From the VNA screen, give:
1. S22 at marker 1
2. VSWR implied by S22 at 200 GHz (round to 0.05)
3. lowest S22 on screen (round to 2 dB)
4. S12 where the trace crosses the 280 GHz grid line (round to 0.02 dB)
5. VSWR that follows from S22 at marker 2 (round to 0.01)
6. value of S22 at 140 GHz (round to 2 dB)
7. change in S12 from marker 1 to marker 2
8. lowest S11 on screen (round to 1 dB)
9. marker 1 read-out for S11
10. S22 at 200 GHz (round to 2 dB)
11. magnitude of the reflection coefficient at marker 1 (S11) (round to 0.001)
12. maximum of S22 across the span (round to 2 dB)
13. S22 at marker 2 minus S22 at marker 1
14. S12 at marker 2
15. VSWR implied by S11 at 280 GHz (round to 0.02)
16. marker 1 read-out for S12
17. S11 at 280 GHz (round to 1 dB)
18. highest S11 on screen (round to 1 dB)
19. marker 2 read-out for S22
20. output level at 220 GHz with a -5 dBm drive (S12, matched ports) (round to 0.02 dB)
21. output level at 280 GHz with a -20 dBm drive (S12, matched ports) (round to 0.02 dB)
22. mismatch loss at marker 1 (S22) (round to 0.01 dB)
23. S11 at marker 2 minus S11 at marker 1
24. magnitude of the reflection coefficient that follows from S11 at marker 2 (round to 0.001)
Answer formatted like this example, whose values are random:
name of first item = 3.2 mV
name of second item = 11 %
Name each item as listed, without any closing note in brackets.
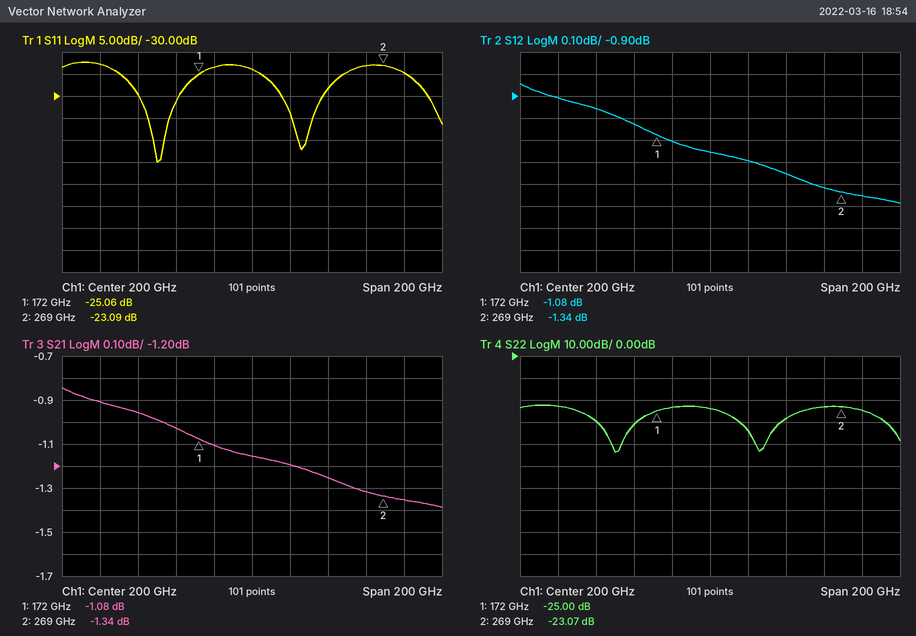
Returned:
S22 at marker 1 = -25.00 dB
VSWR implied by S22 at 200 GHz = 1.15
lowest S22 on screen = -44 dB
S12 where the trace crosses the 280 GHz grid line = -1.36 dB
VSWR that follows from S22 at marker 2 = 1.15
value of S22 at 140 GHz = -30 dB
change in S12 from marker 1 to marker 2 = -0.26 dB
lowest S11 on screen = -45 dB
marker 1 read-out for S11 = -25.06 dB
S22 at 200 GHz = -24 dB
magnitude of the reflection coefficient at marker 1 (S11) = 0.056
maximum of S22 across the span = -22 dB
S22 at marker 2 minus S22 at marker 1 = 1.93 dB
S12 at marker 2 = -1.34 dB
VSWR implied by S11 at 280 GHz = 1.12
marker 1 read-out for S12 = -1.08 dB
S11 at 280 GHz = -25 dB
highest S11 on screen = -22 dB
marker 2 read-out for S22 = -23.07 dB
output level at 220 GHz with a -5 dBm drive (S12, matched ports) = -6.20 dBm
output level at 280 GHz with a -20 dBm drive (S12, matched ports) = -21.36 dBm
mismatch loss at marker 1 (S22) = 0.01 dB
S11 at marker 2 minus S11 at marker 1 = 1.97 dB
magnitude of the reflection coefficient that follows from S11 at marker 2 = 0.070
